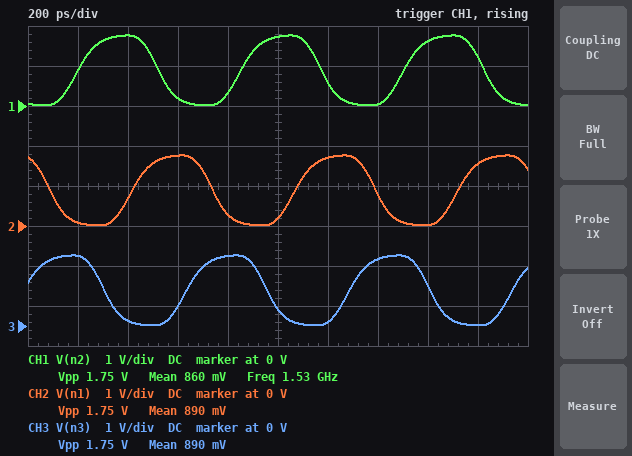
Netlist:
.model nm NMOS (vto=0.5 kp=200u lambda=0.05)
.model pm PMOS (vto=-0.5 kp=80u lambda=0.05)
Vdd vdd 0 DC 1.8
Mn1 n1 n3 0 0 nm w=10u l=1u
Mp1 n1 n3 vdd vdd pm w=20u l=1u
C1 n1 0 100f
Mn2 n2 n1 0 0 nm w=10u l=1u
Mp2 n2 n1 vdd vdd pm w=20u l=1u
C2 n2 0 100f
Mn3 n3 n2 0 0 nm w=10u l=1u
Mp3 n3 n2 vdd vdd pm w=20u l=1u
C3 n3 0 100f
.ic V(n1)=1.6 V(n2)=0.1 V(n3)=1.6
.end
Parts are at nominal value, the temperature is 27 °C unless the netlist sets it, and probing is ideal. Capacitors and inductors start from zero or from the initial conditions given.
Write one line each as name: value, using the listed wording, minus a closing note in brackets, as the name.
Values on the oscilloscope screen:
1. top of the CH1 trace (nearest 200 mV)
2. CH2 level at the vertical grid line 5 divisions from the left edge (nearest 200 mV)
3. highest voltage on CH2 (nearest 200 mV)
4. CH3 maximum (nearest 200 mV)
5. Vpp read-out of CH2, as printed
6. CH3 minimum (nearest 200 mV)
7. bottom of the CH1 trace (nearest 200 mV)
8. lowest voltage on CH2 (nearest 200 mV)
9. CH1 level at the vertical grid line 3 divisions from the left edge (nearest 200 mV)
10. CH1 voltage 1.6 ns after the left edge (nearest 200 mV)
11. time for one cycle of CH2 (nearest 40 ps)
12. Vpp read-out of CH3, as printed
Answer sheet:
top of the CH1 trace: 1.8 V
CH2 level at the vertical grid line 5 divisions from the left edge: 200 mV
highest voltage on CH2: 1.8 V
CH3 maximum: 1.8 V
Vpp read-out of CH2, as printed: 1.75 V
CH3 minimum: 0 V
bottom of the CH1 trace: 0 V
lowest voltage on CH2: 0 V
CH1 level at the vertical grid line 3 divisions from the left edge: 200 mV
CH1 voltage 1.6 ns after the left edge: 1.6 V
time for one cycle of CH2: 640 ps
Vpp read-out of CH3, as printed: 1.75 V
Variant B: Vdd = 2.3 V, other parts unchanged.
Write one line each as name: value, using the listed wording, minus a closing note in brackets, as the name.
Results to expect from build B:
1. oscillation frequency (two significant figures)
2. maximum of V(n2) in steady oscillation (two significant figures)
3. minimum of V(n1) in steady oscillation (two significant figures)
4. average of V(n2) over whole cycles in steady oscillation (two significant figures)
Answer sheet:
oscillation frequency: 2.4 GHz
maximum of V(n2) in steady oscillation: 2.2 V
minimum of V(n1) in steady oscillation: 34 mV
average of V(n2) over whole cycles in steady oscillation: 1.1 V
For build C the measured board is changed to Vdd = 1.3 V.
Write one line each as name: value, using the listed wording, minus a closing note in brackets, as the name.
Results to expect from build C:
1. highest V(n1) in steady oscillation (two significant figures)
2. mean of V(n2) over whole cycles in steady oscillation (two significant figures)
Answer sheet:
highest V(n1) in steady oscillation: 1.3 V
mean of V(n2) over whole cycles in steady oscillation: 640 mV
